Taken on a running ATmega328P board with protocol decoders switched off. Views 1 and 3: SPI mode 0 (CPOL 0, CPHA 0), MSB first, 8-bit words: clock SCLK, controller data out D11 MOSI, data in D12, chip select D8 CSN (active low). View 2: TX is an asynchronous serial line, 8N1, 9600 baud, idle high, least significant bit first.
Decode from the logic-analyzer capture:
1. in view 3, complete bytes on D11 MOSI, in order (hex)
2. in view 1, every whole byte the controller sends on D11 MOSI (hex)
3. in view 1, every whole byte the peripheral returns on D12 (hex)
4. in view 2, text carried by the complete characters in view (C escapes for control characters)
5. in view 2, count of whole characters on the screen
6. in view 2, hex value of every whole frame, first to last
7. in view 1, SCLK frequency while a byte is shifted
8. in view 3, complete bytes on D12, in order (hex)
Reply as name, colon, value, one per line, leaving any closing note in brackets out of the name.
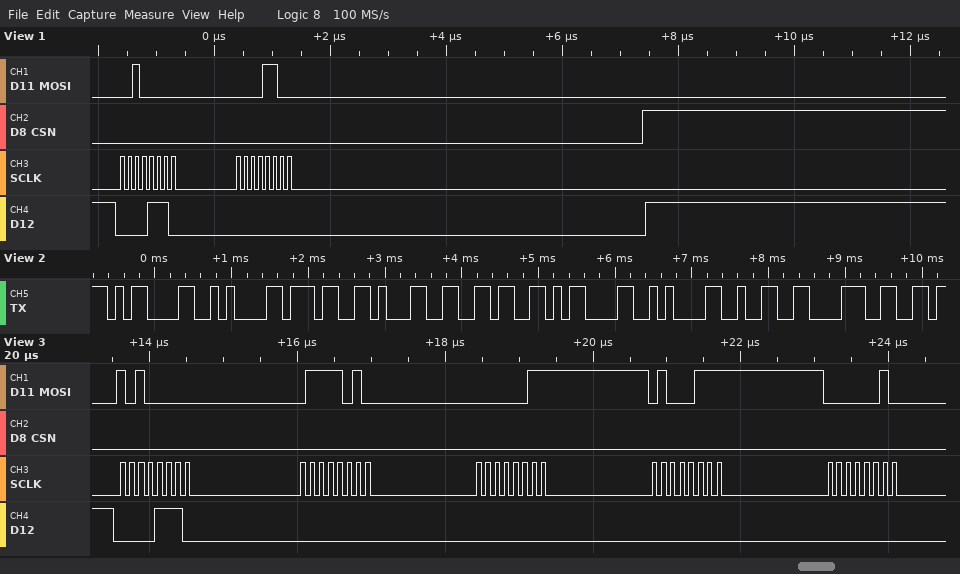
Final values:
in view 3, complete bytes on D11 MOSI, in order: 0xA0 0x7A 0x03 0x47 0x02
in view 1, every whole byte the controller sends on D11 MOSI: 0x20 0x0C
in view 1, every whole byte the peripheral returns on D12: 0x0E 0x00
in view 2, text carried by the complete characters in view: "\r\n716\r\n28"
in view 2, count of whole characters on the screen: 9
in view 2, hex value of every whole frame, first to last: 0D 0A 37 31 36 0D 0A 32 38
in view 1, SCLK frequency while a byte is shifted: 8 MHz
in view 3, complete bytes on D12, in order: 0x0E 0x00 0x00 0x00 0x00
